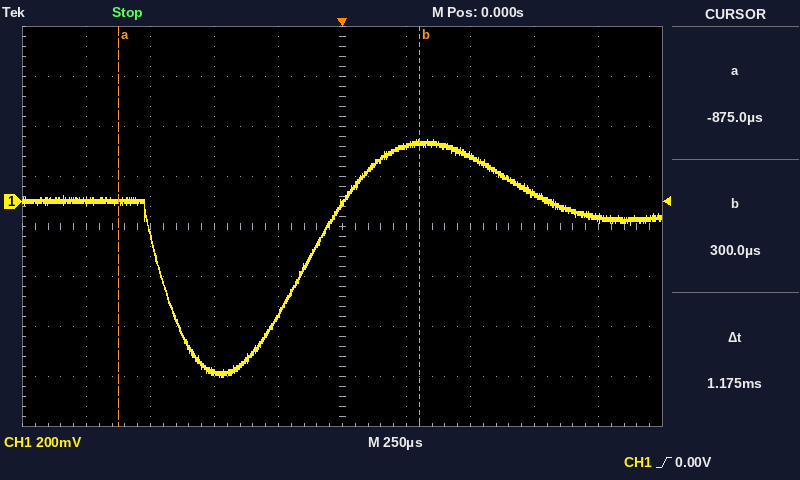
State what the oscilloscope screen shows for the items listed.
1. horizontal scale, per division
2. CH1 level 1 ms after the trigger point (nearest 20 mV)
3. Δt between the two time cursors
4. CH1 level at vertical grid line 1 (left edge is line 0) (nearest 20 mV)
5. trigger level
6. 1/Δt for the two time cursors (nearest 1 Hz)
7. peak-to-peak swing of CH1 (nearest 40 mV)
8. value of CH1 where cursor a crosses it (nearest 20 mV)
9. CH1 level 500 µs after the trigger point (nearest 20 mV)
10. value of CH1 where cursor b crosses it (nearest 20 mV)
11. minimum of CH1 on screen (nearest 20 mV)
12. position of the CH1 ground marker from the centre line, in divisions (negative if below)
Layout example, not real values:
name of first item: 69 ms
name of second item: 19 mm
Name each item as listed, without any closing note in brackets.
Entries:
horizontal scale, per division: 250 µs
CH1 level 1 ms after the trigger point: -60 mV
Δt between the two time cursors: 1.175 ms
CH1 level at vertical grid line 1 (left edge is line 0): 0 mV
trigger level: 0.00 V
1/Δt for the two time cursors: 851 Hz
peak-to-peak swing of CH1: 960 mV
value of CH1 where cursor a crosses it: 0 mV
CH1 level 500 µs after the trigger point: 180 mV
value of CH1 where cursor b crosses it: 240 mV
minimum of CH1 on screen: -700 mV
position of the CH1 ground marker from the centre line, in divisions: +0.5 div
